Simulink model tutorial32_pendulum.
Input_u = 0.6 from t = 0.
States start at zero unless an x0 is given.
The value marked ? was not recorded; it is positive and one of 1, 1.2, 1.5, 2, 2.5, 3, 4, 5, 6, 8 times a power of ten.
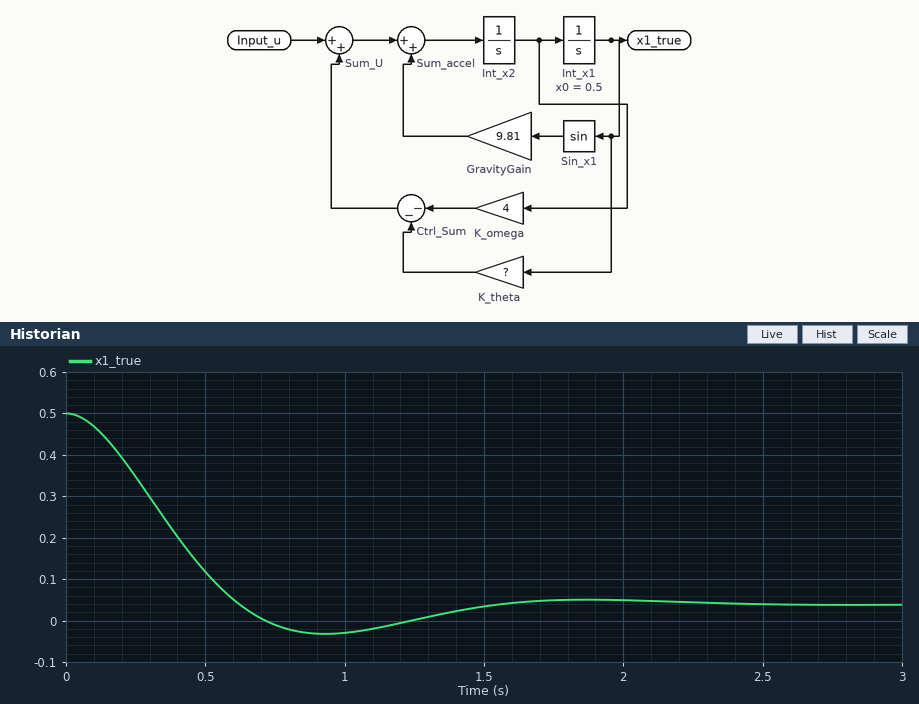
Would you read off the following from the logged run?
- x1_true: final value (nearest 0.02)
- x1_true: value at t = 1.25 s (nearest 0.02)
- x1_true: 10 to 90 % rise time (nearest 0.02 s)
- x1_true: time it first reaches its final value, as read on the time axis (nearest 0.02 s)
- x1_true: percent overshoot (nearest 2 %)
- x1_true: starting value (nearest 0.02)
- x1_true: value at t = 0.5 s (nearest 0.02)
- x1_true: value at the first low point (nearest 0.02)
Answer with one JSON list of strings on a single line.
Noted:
["0.04", "0.00", "0.42 s", "0.62 s", "16 %", "0.50", "0.12", "-0.04"]
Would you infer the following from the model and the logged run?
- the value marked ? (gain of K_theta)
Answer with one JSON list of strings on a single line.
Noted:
["25"]
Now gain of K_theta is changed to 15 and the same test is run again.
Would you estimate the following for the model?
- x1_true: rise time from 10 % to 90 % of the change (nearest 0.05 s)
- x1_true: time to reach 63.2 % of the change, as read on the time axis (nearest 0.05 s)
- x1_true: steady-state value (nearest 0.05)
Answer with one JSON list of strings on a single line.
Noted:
["1.15 s", "0.80 s", "0.10"]
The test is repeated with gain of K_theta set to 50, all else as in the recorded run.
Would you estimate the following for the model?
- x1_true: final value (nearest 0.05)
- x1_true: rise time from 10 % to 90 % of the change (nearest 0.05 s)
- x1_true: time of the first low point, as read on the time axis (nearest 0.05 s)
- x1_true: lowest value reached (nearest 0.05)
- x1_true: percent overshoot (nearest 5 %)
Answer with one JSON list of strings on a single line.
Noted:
["0.00", "0.20 s", "0.50 s", "-0.15", "35 %"]
